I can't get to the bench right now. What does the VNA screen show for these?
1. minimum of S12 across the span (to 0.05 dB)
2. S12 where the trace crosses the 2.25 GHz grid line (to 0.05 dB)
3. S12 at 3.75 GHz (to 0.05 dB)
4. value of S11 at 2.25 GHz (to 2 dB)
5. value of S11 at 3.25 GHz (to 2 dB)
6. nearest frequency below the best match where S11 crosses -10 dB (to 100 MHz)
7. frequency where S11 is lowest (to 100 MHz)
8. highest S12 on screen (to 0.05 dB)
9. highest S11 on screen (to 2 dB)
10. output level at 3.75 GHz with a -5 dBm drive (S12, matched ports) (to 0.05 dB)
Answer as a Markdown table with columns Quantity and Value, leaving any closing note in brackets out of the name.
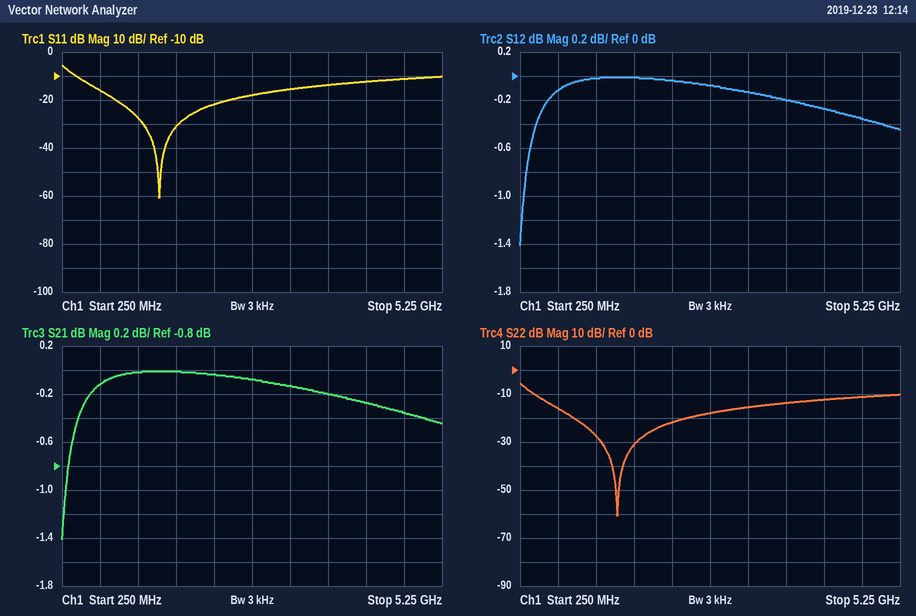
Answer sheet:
| Quantity | Value |
|---|---|
| minimum of S12 across the span | -1.40 dB |
| S12 where the trace crosses the 2.25 GHz grid line | -0.05 dB |
| S12 at 3.75 GHz | -0.20 dB |
| value of S11 at 2.25 GHz | -22 dB |
| value of S11 at 3.25 GHz | -16 dB |
| nearest frequency below the best match where S11 crosses -10 dB | 400 MHz |
| frequency where S11 is lowest | 1.5 GHz |
| highest S12 on screen | 0.00 dB |
| highest S11 on screen | -6 dB |
| output level at 3.75 GHz with a -5 dBm drive (S12, matched ports) | -5.20 dBm |
